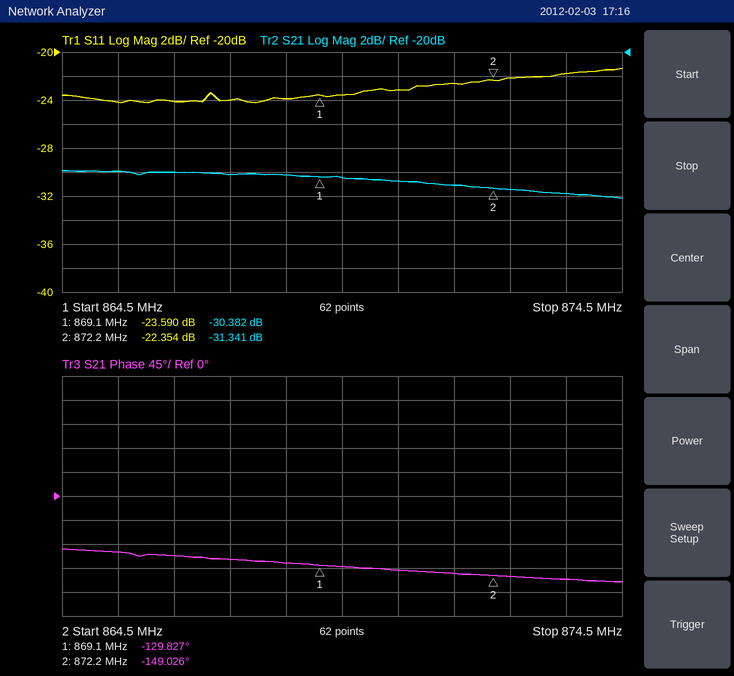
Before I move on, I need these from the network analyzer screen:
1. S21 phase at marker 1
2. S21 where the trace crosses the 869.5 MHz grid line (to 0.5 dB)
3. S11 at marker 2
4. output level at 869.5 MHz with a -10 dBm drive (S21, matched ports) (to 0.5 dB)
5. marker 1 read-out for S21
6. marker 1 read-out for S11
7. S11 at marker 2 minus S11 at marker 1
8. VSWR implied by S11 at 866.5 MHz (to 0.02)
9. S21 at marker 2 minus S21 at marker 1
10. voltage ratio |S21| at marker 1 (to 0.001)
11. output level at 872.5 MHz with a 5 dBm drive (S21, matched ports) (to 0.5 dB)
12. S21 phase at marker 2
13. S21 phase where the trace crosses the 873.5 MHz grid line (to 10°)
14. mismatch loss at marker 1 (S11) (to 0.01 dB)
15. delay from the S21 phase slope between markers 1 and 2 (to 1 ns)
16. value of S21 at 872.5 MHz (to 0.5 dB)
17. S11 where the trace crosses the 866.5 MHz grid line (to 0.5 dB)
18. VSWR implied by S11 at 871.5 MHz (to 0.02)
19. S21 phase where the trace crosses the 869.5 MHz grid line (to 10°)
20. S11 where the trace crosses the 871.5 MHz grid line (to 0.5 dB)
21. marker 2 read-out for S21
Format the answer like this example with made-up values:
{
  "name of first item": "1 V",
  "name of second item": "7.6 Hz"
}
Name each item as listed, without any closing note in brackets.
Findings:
{
  "S21 phase at marker 1": "-129.827°",
  "S21 where the trace crosses the 869.5 MHz grid line": "-30.5 dB",
  "S11 at marker 2": "-22.354 dB",
  "output level at 869.5 MHz with a -10 dBm drive (S21, matched ports)": "-40.5 dBm",
  "marker 1 read-out for S21": "-30.382 dB",
  "marker 1 read-out for S11": "-23.590 dB",
  "S11 at marker 2 minus S11 at marker 1": "1.236 dB",
  "VSWR implied by S11 at 866.5 MHz": "1.14",
  "S21 at marker 2 minus S21 at marker 1": "-0.959 dB",
  "voltage ratio |S21| at marker 1": "0.030",
  "output level at 872.5 MHz with a 5 dBm drive (S21, matched ports)": "-26.5 dBm",
  "S21 phase at marker 2": "-149.026°",
  "S21 phase where the trace crosses the 873.5 MHz grid line": "-160°",
  "mismatch loss at marker 1 (S11)": "0.02 dB",
  "delay from the S21 phase slope between markers 1 and 2": "17 ns",
  "value of S21 at 872.5 MHz": "-31.5 dB",
  "S11 where the trace crosses the 866.5 MHz grid line": "-24.0 dB",
  "VSWR implied by S11 at 871.5 MHz": "1.16",
  "S21 phase where the trace crosses the 869.5 MHz grid line": "-130°",
  "S11 where the trace crosses the 871.5 MHz grid line": "-22.5 dB",
  "marker 2 read-out for S21": "-31.341 dB"
}
